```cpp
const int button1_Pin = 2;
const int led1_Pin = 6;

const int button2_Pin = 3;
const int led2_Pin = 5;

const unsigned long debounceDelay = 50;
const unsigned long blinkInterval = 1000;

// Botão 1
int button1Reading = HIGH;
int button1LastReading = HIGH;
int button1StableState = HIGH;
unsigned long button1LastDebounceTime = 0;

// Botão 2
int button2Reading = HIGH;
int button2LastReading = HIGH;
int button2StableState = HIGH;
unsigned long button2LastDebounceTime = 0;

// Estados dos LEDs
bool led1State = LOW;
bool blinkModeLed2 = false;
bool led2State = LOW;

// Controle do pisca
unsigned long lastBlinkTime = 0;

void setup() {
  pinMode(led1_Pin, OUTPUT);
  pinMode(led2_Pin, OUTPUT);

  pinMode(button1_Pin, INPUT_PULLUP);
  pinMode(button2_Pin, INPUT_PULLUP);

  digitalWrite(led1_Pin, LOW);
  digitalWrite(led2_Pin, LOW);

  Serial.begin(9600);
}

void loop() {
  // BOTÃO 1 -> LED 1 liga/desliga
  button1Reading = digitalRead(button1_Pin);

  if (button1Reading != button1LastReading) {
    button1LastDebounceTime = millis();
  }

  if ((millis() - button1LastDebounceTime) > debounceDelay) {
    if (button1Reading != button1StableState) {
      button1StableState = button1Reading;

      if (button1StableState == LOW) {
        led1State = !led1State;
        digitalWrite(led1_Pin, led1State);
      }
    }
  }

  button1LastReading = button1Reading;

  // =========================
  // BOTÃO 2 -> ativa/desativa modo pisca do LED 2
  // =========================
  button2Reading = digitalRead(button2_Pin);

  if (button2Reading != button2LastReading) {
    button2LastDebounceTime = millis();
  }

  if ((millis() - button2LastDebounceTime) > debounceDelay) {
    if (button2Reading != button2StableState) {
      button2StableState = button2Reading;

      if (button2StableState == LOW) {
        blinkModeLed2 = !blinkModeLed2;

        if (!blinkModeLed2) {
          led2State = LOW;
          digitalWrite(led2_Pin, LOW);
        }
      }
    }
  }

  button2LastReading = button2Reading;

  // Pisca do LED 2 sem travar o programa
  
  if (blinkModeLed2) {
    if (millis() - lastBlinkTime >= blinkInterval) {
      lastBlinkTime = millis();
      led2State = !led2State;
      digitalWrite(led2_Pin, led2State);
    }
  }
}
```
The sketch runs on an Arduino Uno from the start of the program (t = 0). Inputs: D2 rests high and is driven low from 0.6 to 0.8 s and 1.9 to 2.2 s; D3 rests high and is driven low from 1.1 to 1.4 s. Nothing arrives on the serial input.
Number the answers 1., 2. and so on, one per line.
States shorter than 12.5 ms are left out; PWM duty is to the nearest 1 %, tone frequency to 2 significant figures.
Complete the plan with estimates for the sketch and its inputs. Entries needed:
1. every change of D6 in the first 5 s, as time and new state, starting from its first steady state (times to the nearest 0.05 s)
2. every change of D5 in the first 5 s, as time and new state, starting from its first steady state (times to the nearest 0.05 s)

1. 0 s low; 0.65 s high; 1.95 s low
2. 0 s low; 1.15 s high; 2.15 s low; 3.15 s high; 4.15 s low
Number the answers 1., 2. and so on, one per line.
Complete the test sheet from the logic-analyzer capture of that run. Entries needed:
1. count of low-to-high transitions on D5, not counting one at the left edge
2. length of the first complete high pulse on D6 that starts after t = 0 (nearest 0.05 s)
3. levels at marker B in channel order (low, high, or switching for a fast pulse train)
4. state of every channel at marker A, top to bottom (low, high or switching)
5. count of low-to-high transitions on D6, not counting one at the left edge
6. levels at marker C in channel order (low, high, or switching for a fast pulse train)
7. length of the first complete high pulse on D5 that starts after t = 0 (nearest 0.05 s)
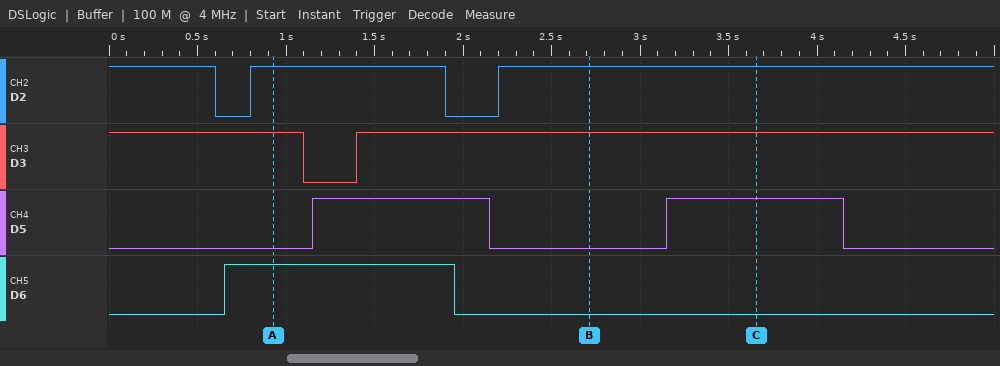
1. 2
2. 1.30 s
3. D2 high, D3 high, D5 low, D6 low
4. D2 high, D3 high, D5 low, D6 high
5. 1
6. D2 high, D3 high, D5 high, D6 low
7. 1.00 s
